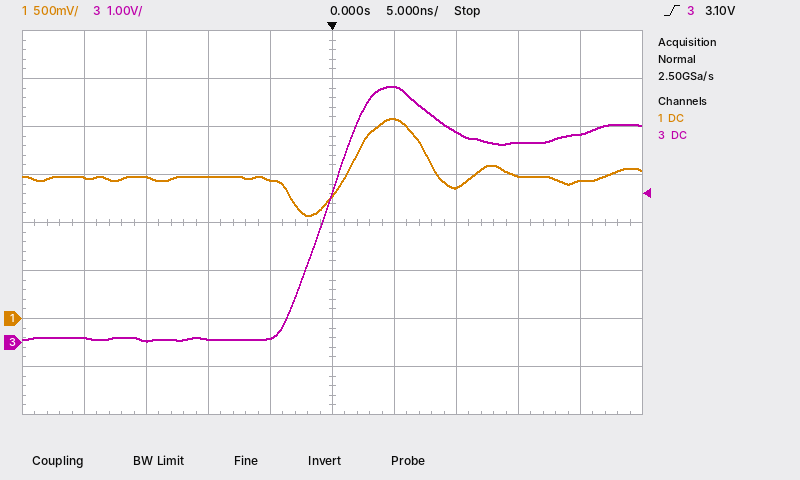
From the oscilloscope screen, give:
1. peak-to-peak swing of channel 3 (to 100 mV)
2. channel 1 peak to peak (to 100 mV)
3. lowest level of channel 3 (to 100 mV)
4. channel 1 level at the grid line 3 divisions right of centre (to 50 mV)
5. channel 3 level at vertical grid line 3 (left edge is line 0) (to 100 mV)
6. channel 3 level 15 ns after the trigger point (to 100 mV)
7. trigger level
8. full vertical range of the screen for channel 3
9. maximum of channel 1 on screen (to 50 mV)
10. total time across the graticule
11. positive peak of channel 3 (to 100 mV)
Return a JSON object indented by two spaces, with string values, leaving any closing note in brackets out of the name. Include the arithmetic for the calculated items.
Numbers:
{
  "peak-to-peak swing of channel 3": "5.3 V − (0.0 V) = 5.3 V",
  "channel 1 peak to peak": "1.00 V",
  "lowest level of channel 3": "0.0 V",
  "channel 1 level at the grid line 3 divisions right of centre": "1.50 V",
  "channel 3 level at vertical grid line 3 (left edge is line 0)": "100 mV",
  "channel 3 level 15 ns after the trigger point": "4.2 V",
  "trigger level": "3.10 V",
  "full vertical range of the screen for channel 3": "8 V",
  "maximum of channel 1 on screen": "2.10 V",
  "total time across the graticule": "50 ns",
  "positive peak of channel 3": "5.3 V"
}
